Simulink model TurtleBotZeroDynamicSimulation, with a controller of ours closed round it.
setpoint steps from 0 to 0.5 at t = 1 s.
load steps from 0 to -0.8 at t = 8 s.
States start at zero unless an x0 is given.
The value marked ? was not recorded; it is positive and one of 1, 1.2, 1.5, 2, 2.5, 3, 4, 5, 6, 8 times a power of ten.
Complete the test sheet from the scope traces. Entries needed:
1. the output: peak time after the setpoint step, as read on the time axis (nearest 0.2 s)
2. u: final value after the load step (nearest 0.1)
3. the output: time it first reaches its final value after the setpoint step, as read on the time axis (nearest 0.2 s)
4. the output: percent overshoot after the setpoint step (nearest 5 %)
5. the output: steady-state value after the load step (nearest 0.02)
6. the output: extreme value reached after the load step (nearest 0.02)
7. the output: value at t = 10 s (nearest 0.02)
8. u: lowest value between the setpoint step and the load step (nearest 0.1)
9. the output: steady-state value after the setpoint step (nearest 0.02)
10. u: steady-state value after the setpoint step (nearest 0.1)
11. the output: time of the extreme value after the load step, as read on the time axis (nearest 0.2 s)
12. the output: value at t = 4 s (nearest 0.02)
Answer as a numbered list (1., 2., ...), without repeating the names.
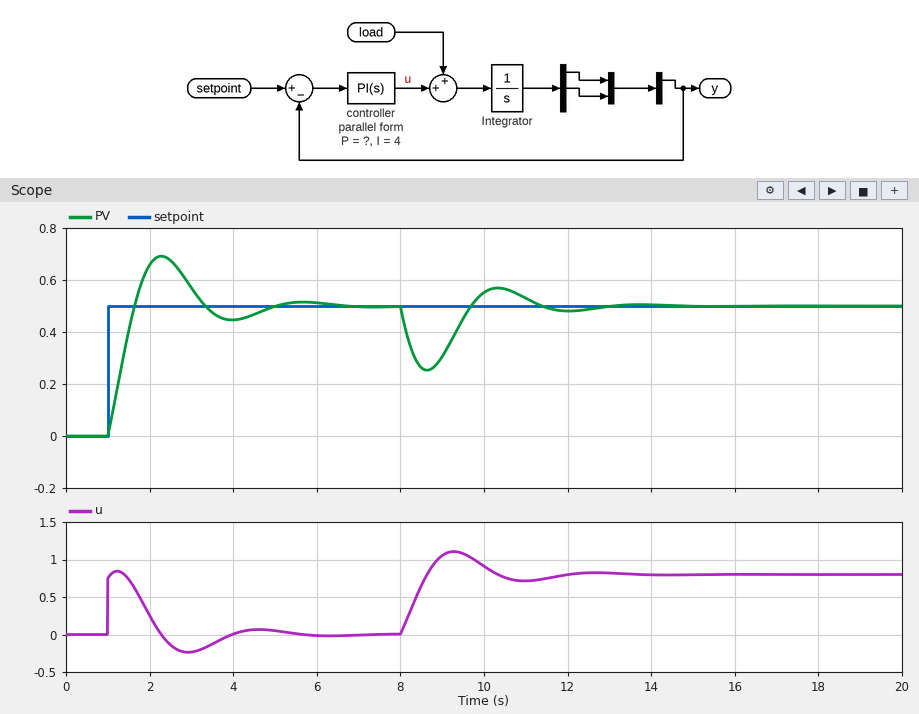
1. 2.2 s
2. 0.8
3. 1.6 s
4. 40 %
5. 0.50
6. 0.26
7. 0.56
8. -0.2
9. 0.50
10. 0.0
11. 8.6 s
12. 0.44
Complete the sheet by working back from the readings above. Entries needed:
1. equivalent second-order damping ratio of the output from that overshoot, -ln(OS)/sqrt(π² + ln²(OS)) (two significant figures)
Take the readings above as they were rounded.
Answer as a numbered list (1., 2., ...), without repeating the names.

1. 0.28
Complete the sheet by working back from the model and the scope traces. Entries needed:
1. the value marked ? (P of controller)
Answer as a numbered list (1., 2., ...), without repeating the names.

1. 1.5
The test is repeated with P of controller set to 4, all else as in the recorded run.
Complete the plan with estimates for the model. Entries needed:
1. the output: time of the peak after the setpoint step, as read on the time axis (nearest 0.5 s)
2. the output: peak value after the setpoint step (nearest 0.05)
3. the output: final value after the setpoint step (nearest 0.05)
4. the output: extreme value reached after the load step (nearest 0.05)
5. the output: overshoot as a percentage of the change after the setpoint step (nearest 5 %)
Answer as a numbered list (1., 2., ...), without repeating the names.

1. 2.0 s
2. 0.55
3. 0.50
4. 0.35
5. 15 %
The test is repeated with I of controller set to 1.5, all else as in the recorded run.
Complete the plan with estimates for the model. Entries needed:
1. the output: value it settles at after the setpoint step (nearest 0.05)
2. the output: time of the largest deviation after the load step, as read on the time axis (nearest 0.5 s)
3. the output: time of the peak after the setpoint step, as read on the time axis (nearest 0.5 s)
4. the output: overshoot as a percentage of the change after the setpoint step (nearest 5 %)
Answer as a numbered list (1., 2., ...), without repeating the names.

1. 0.50
2. 9.0 s
3. 3.0 s
4. 25 %
